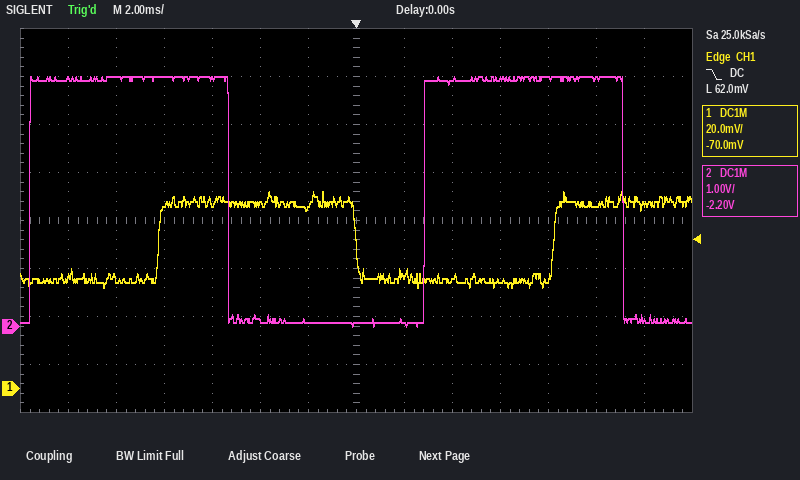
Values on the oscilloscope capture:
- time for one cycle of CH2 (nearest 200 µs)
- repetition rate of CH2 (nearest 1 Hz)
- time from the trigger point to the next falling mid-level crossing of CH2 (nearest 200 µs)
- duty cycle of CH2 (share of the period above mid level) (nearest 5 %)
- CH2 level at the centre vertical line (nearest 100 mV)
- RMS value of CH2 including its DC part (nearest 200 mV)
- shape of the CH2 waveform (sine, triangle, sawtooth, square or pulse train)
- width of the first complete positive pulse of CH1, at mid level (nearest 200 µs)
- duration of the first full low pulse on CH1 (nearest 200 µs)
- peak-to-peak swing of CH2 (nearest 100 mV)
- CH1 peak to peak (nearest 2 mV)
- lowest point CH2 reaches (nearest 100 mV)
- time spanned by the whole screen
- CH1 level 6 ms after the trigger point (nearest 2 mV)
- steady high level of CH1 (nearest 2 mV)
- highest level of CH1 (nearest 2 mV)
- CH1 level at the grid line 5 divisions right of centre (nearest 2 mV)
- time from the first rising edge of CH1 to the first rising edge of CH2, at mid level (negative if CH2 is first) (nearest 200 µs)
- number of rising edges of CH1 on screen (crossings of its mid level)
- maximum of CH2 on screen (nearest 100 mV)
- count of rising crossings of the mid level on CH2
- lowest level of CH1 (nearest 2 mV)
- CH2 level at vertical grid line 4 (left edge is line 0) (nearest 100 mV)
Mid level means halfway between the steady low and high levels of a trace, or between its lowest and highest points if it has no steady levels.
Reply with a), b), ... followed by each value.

a) 16.4 ms
b) 61 Hz
c) 11.2 ms
d) 50 %
e) 100 mV
f) 3.6 V
g) square
h) 8.2 ms
i) 8.2 ms
j) 5.2 V
k) 40 mV
l) 0.0 V
m) 28 ms
n) 44 mV
o) 78 mV
p) 82 mV
q) 76 mV
r) -5.4 ms
s) 2
t) 5.2 V
u) 2
v) 42 mV
w) 5.2 V
